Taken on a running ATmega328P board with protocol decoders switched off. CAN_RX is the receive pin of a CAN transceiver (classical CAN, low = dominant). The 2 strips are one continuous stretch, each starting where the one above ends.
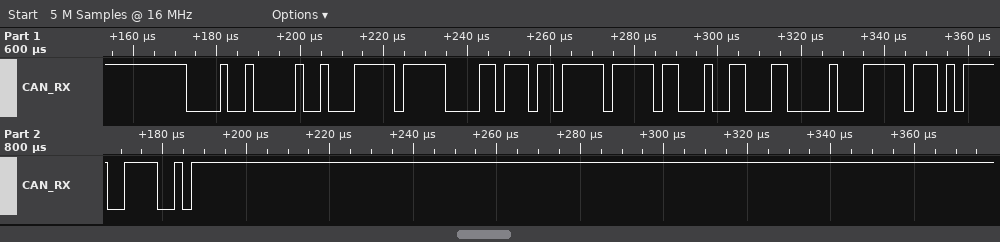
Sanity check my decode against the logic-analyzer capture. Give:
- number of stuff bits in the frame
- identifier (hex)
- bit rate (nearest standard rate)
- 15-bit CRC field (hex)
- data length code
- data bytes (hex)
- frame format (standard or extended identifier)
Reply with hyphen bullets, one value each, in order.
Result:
- 7
- 0x090
- 500 kbit/s
- 0x2F3C
- 8
- FF C6 ED FF E2 63 00 FF
- standard
